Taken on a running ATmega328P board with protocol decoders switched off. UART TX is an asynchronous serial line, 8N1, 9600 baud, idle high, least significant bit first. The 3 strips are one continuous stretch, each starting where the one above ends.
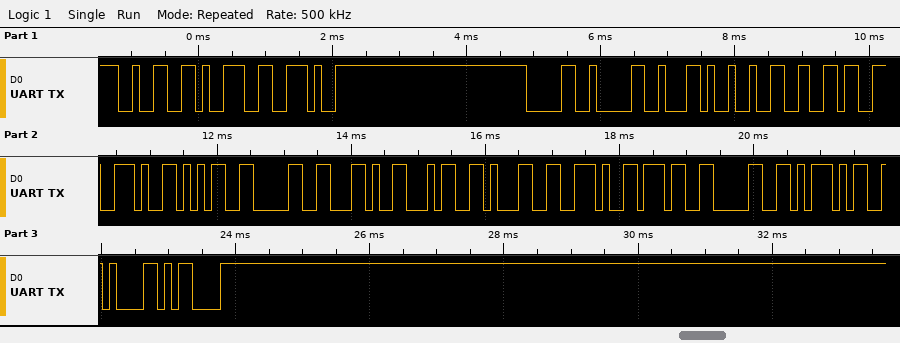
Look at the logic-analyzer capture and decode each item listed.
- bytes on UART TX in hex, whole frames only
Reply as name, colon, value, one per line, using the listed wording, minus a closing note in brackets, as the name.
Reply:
bytes on UART TX in hex, whole frames only: 32 39 2E 30 30 2C 32 36 2E 35 30 2C 34 31 2E 37 30 5D 0A 0D
